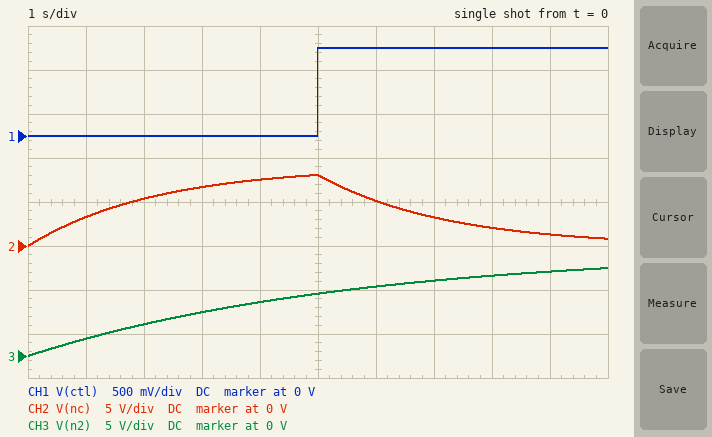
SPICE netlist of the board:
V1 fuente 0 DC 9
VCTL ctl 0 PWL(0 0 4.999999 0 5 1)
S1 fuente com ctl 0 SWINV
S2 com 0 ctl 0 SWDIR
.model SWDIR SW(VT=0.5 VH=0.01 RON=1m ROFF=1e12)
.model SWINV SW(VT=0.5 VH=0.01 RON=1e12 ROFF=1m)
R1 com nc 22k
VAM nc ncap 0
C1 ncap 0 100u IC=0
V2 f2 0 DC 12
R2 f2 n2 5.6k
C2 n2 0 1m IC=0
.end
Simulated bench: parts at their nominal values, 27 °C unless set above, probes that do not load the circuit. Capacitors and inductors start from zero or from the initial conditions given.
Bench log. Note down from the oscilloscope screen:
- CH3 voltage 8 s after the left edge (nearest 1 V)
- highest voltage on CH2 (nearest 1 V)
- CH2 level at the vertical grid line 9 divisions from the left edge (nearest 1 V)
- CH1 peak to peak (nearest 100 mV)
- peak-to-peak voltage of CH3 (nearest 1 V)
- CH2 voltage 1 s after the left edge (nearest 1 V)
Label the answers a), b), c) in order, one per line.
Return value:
a) 9 V
b) 8 V
c) 1 V
d) 1.0 V
e) 10 V
f) 3 V
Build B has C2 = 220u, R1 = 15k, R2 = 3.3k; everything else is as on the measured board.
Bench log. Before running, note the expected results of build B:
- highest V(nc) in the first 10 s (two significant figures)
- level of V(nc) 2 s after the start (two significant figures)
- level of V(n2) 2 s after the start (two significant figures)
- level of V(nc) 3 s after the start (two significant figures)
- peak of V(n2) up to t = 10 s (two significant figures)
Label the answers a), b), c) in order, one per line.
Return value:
a) 8.7 V
b) 6.6 V
c) 11 V
d) 7.8 V
e) 12 V
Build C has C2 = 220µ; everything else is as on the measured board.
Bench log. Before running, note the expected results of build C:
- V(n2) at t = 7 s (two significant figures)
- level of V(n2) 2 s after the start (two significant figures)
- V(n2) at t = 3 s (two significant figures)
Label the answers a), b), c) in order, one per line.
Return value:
a) 12 V
b) 9.6 V
c) 11 V
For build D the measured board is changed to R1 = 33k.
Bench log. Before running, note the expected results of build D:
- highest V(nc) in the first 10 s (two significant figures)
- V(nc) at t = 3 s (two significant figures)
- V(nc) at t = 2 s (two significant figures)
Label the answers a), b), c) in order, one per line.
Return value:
a) 7.0 V
b) 5.4 V
c) 4.1 V
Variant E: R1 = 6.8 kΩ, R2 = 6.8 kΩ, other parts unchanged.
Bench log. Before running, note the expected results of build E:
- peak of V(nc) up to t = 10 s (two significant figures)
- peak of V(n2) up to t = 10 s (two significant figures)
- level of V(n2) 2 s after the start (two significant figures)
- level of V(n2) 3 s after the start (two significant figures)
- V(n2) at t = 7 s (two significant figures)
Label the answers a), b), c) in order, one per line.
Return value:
a) 9.0 V
b) 9.2 V
c) 3.1 V
d) 4.3 V
e) 7.7 V
